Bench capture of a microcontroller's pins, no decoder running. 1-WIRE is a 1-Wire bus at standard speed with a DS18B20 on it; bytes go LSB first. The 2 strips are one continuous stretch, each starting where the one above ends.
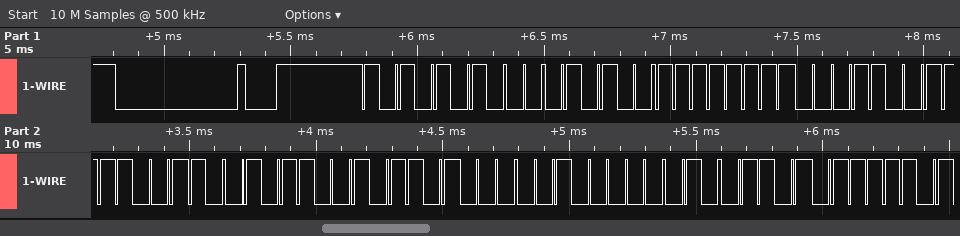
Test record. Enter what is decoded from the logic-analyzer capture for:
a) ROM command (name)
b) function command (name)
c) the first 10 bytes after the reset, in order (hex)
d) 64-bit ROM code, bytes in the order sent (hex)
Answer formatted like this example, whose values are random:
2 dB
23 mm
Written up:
Match ROM
Read Scratchpad
55 28 FF 98 67 9A 16 04 B2 BE
28 FF 98 67 9A 16 04 B2
